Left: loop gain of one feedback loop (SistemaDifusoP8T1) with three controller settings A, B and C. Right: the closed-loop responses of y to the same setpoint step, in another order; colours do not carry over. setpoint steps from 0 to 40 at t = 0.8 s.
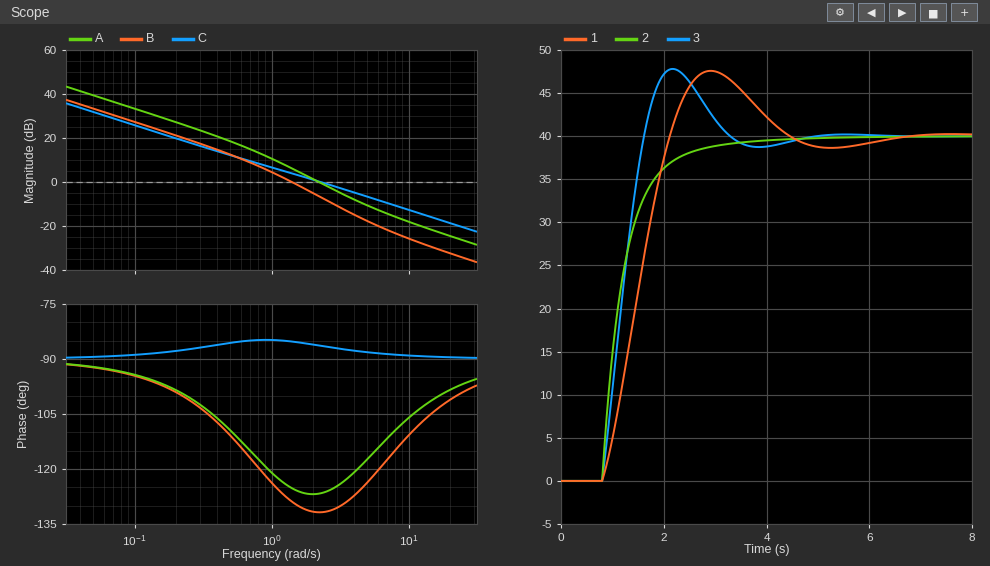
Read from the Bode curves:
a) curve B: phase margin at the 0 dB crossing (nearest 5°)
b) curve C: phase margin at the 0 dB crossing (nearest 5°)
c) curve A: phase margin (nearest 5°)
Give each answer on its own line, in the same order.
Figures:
50°
95°
55°
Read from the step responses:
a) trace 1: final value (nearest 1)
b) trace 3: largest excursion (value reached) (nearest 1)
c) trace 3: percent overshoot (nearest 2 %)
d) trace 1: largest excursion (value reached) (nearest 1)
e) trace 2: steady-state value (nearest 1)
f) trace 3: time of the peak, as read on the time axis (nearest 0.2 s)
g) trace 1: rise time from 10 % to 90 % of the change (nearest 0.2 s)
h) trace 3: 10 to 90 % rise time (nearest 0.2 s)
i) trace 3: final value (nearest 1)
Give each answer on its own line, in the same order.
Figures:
40
48
20 %
48
40
2.2 s
1.0 s
0.6 s
40
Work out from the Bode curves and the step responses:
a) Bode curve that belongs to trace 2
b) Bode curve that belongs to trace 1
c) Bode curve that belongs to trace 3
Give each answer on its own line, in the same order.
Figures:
C
B
A
